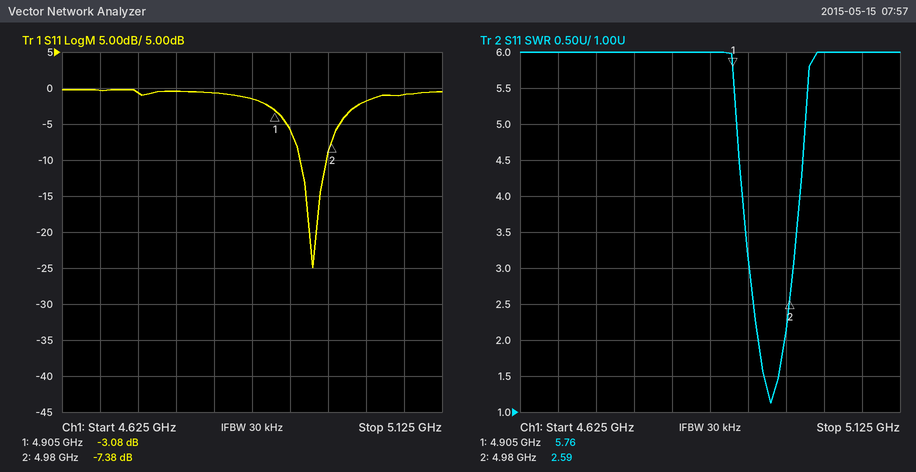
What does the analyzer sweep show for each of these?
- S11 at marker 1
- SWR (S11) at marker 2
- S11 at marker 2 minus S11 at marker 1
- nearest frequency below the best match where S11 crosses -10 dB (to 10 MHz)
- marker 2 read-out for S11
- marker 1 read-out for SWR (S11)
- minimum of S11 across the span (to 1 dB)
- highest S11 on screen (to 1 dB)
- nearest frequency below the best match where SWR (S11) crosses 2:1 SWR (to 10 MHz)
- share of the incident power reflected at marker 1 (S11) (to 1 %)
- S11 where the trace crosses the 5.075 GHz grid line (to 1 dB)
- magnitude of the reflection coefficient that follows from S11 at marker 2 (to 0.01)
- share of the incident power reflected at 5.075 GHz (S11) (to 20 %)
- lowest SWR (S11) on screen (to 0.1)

-3.08 dB
2.59
-4.30 dB
4.94 GHz
-7.38 dB
5.76
-25 dB
0 dB
4.94 GHz
49 %
-1 dB
0.43
80 %
1.1
